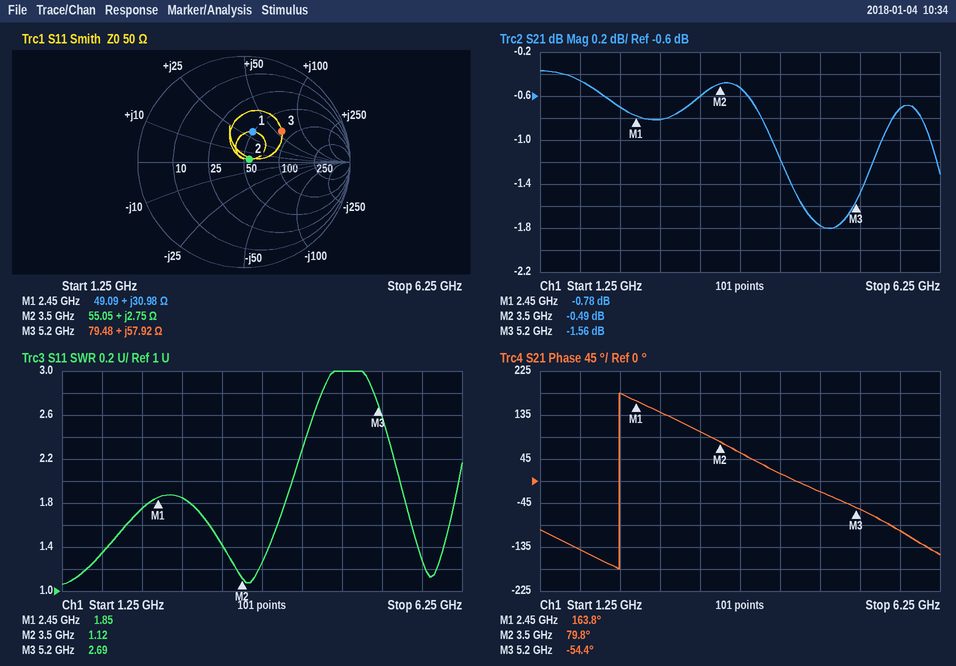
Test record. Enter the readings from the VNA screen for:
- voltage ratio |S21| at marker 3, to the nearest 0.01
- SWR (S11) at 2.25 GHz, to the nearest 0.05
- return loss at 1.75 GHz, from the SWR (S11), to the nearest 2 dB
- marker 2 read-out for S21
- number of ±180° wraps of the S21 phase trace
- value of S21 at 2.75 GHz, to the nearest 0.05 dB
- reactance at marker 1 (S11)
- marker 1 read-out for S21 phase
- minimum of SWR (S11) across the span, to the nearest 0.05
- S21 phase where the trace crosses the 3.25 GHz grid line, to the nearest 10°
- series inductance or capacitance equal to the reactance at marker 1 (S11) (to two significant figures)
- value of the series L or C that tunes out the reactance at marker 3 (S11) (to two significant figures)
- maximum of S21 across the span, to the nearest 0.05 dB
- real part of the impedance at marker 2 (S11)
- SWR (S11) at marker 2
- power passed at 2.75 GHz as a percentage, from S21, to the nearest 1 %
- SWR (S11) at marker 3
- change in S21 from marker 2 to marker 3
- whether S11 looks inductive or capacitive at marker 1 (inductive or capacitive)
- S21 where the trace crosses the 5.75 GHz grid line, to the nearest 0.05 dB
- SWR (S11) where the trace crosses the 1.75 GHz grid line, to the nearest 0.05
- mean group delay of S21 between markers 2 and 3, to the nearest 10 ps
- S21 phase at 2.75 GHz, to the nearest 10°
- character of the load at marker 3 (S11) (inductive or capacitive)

0.84
1.75
16 dB
-0.49 dB
1
-0.80 dB
+30.98 Ω
163.8°
1.05
100°
2.0 nH
530 fF
-0.35 dB
55.05 Ω
1.12
83 %
2.69
-1.07 dB
inductive
-0.70 dB
1.35
220 ps
140°
inductive
